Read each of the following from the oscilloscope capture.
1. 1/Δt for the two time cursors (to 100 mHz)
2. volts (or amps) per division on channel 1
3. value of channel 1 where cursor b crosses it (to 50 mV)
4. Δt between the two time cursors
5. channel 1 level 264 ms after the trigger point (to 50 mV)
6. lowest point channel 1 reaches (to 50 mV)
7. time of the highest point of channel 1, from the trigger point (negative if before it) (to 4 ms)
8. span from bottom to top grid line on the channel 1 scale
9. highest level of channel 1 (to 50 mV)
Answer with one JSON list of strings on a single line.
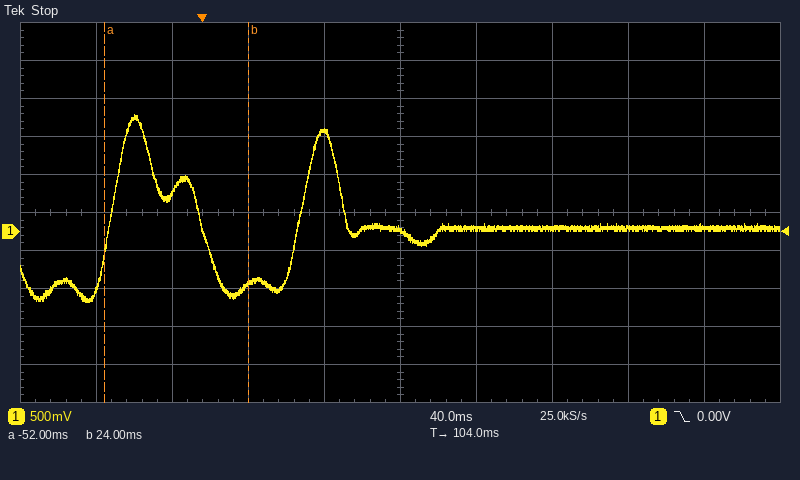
["13.2 Hz", "500 mV", "-700 mV", "76 ms", "50 mV", "-950 mV", "-36 ms", "5 V", "1.55 V"]
